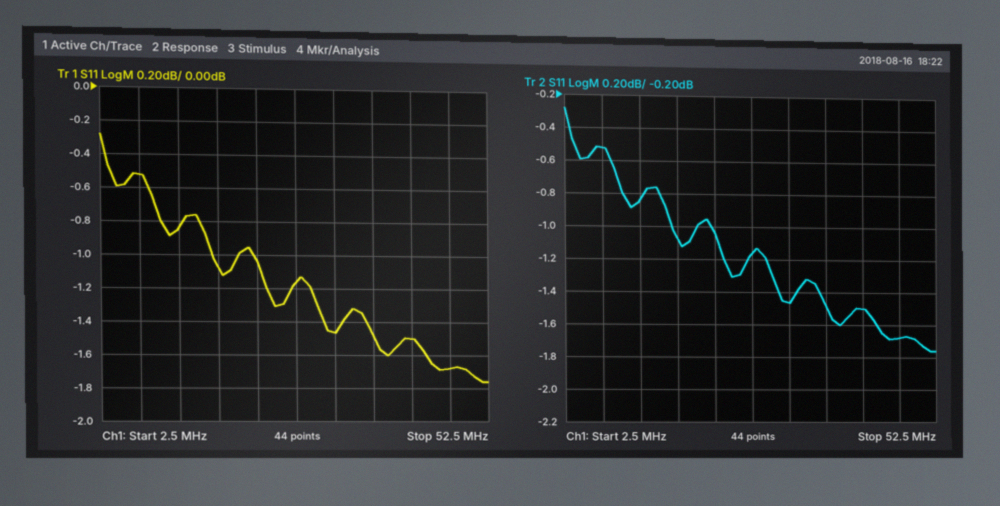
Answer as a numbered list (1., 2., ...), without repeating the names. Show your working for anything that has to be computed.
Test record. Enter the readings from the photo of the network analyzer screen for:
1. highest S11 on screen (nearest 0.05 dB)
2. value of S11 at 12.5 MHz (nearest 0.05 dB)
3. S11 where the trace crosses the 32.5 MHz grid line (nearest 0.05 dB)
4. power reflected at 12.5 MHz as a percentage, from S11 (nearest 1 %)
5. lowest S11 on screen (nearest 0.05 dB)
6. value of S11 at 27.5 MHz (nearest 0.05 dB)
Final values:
1. -0.30 dB
2. -0.85 dB
3. -1.45 dB
4. 10^(-0.85/10) ≈ 82 %
5. -1.75 dB
6. -1.15 dB
